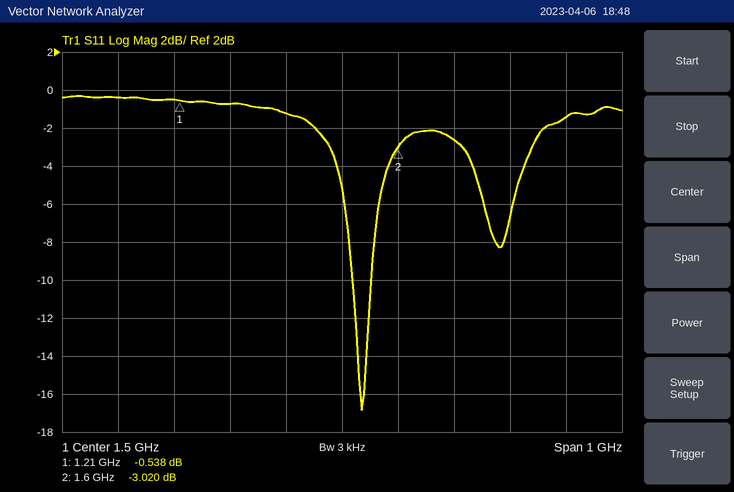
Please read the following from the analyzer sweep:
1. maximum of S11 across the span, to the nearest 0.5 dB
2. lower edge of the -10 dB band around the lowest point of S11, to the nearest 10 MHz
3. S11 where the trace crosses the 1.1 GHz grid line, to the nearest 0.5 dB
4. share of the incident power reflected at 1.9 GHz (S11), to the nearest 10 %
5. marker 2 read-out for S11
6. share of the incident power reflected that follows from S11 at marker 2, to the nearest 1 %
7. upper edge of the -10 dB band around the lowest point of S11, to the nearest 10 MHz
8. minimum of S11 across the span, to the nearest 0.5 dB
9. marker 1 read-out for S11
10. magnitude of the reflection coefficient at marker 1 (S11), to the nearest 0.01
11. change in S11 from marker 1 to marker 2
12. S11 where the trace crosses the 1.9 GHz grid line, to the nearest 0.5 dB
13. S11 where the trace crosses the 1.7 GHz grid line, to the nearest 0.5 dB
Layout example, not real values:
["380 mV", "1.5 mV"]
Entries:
["-0.5 dB", "1.52 GHz", "-0.5 dB", "70 %", "-3.020 dB", "50 %", "1.55 GHz", "-17.0 dB", "-0.538 dB", "0.94", "-2.482 dB", "-1.5 dB", "-2.5 dB"]
